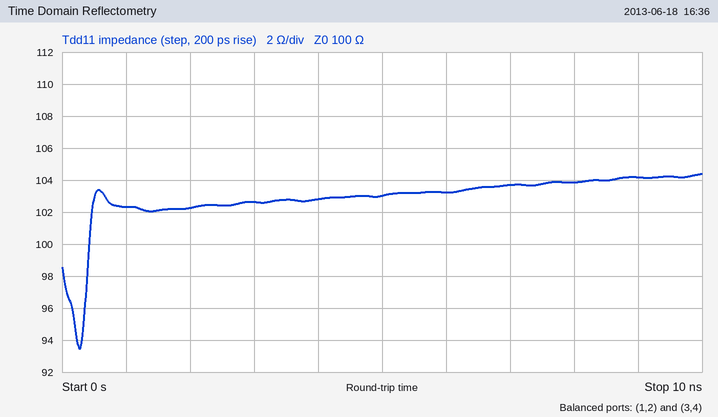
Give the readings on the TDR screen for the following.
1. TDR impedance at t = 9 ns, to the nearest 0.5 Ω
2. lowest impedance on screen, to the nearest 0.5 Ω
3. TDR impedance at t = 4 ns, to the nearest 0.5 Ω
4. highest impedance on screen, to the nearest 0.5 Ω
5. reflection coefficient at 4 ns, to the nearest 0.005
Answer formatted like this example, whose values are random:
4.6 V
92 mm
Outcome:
104.0 Ω
93.5 Ω
103.0 Ω
104.5 Ω
+0.015
